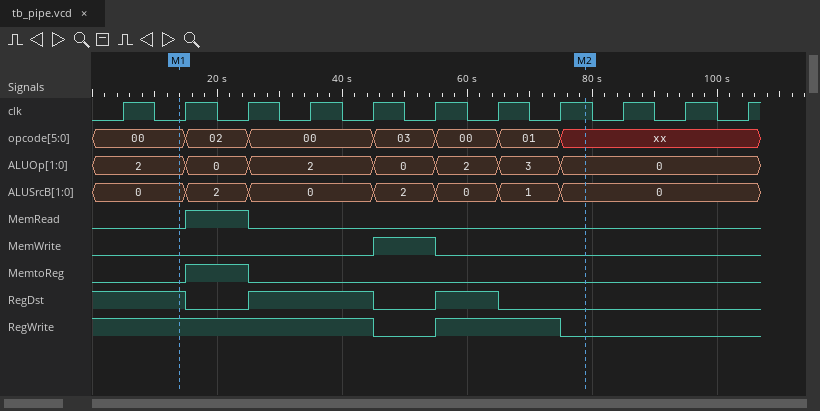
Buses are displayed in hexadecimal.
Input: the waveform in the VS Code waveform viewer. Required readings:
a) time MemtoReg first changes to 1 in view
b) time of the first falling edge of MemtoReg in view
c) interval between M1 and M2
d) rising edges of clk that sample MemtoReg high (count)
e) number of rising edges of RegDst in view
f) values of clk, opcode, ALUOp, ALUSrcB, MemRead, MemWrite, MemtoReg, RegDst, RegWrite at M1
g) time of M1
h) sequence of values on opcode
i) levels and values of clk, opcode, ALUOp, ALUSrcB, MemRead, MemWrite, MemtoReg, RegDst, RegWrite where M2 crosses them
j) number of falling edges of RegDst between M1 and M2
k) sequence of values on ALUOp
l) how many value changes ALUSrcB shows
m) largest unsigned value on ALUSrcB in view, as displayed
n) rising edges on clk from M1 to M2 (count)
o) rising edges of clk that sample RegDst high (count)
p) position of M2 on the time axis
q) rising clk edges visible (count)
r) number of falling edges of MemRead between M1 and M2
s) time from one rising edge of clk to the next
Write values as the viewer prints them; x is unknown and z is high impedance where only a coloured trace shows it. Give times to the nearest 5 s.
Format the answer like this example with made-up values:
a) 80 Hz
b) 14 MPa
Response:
a) 15 s
b) 25 s
c) 65 s
d) 1
e) 2
f) clk=0, opcode=00, ALUOp=2, ALUSrcB=0, MemRead=0, MemWrite=0, MemtoReg=0, RegDst=1, RegWrite=1
g) 15 s
h) 00, 02, 00, 03, 00, 01, xx
i) clk=1, opcode=xx, ALUOp=0, ALUSrcB=0, MemRead=0, MemWrite=0, MemtoReg=0, RegDst=0, RegWrite=0
j) 3
k) 2, 0, 2, 0, 2, 3, 0
l) 6
m) 2
n) 7
o) 5
p) 80 s
q) 11
r) 1
s) 10 s
